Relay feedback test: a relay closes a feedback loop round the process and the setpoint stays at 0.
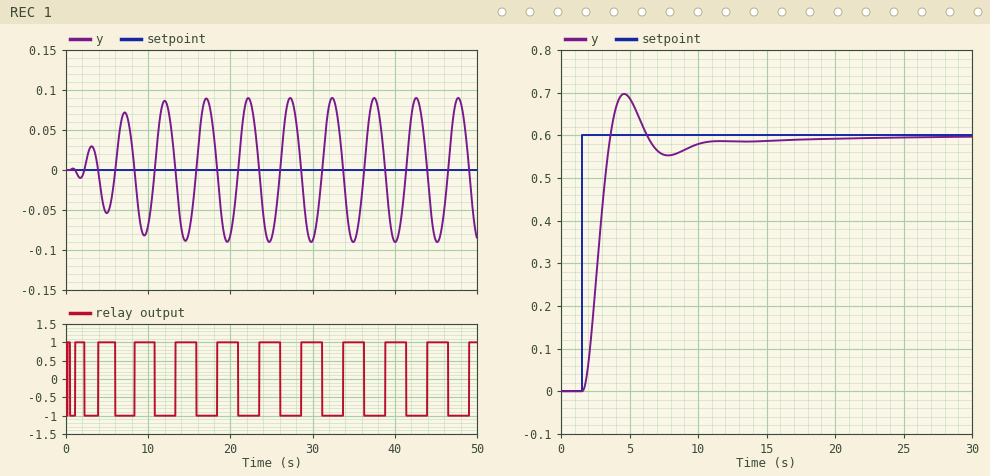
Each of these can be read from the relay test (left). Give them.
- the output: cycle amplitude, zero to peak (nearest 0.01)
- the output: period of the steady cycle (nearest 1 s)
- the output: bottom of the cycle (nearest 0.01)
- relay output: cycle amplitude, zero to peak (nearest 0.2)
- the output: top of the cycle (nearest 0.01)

0.09
5 s
-0.09
1.0
0.09
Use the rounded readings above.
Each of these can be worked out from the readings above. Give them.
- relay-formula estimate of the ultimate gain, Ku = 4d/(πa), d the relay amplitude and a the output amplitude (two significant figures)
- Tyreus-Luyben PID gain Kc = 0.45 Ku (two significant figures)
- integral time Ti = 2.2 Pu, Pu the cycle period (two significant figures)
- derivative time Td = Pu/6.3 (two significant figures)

14
6.3
11 s
0.79 s
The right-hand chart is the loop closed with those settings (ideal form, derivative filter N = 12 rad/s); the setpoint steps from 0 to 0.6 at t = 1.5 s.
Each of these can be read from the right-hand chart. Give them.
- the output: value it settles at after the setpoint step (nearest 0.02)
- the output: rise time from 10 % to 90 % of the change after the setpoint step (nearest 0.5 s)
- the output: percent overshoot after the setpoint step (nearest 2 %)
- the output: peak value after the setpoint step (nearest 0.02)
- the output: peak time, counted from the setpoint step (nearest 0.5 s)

0.60
1.5 s
16 %
0.70
3.0 s
